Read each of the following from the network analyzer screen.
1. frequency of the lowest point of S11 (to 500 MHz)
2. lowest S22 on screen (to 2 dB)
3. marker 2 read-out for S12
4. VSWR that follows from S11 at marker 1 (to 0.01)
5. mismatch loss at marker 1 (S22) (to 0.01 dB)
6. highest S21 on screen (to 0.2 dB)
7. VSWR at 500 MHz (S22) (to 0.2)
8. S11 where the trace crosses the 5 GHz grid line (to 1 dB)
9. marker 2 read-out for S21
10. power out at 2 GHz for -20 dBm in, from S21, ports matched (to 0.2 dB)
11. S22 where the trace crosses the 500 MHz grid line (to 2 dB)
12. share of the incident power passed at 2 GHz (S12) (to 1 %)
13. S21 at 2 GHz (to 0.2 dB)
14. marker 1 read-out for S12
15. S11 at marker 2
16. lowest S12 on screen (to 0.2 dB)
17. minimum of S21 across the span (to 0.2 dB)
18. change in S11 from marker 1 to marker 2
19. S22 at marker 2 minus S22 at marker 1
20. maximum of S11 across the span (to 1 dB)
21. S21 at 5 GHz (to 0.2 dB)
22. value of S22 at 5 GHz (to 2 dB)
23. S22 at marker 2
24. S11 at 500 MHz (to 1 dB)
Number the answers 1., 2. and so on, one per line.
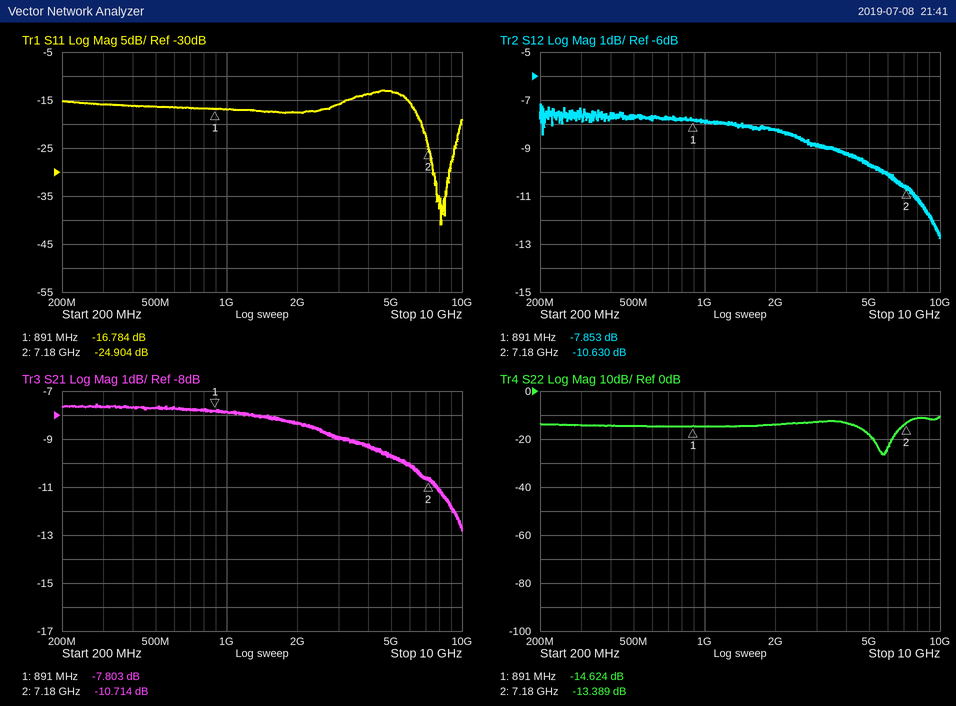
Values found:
1. 8.0 GHz
2. -26 dB
3. -10.630 dB
4. 1.34
5. 0.15 dB
6. -7.6 dB
7. 1.4
8. -13 dB
9. -10.714 dB
10. -28.4 dBm
11. -14 dB
12. 15 %
13. -8.4 dB
14. -7.853 dB
15. -24.904 dB
16. -12.8 dB
17. -12.8 dB
18. -8.120 dB
19. 1.235 dB
20. -13 dB
21. -9.8 dB
22. -18 dB
23. -13.389 dB
24. -16 dB
